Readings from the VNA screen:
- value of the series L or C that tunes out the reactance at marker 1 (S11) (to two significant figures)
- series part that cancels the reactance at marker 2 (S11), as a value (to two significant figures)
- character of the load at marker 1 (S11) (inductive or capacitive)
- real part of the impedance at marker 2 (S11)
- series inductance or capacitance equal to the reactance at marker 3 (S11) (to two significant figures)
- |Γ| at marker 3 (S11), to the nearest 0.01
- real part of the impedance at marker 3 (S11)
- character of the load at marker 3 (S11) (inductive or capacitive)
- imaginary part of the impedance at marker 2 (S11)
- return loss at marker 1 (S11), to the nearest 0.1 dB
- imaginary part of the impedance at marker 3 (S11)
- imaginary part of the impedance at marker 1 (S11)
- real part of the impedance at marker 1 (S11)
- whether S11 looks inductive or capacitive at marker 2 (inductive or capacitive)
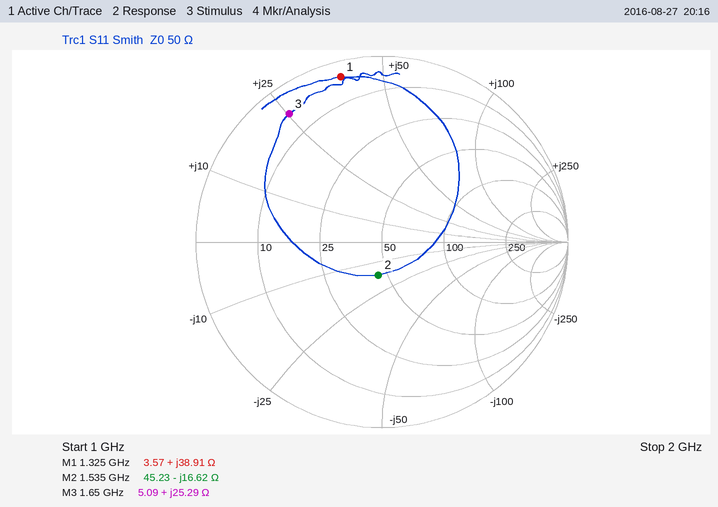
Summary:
3.1 pF
1.7 nH
inductive
45.23 Ω
2.4 nH
0.85
5.09 Ω
inductive
-16.62 Ω
0.8 dB
+25.29 Ω
+38.91 Ω
3.57 Ω
capacitive
